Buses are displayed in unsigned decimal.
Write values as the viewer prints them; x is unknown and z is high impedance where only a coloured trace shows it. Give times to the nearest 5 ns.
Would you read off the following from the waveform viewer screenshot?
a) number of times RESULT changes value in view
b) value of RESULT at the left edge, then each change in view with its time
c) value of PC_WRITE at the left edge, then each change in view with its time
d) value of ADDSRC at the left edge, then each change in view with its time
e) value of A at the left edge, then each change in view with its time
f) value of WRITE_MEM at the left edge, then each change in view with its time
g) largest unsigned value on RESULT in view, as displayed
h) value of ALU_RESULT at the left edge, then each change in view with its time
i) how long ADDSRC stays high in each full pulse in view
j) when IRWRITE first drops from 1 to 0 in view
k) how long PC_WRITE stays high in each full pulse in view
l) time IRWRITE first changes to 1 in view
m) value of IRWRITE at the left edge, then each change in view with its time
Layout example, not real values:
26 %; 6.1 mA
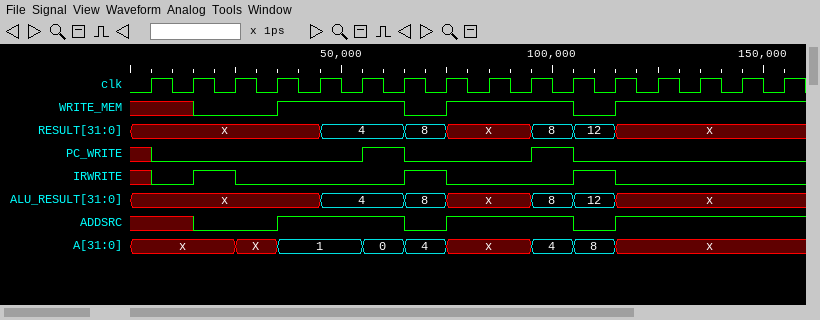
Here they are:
6; x, 4 at 45 ns, 8 at 65 ns, x at 75 ns, 8 at 95 ns, 12 at 105 ns, x at 115 ns; x, 0 at 5 ns, 1 at 55 ns, 0 at 65 ns, 1 at 95 ns, 0 at 105 ns; x, 0 at 15 ns, 1 at 35 ns, 0 at 65 ns, 1 at 75 ns, 0 at 105 ns, 1 at 115 ns; x, X at 25 ns, 1 at 35 ns, 0 at 55 ns, 4 at 65 ns, x at 75 ns, 4 at 95 ns, 8 at 105 ns, x at 115 ns; x, 0 at 15 ns, 1 at 35 ns, 0 at 65 ns, 1 at 75 ns, 0 at 105 ns, 1 at 115 ns; 12; x, 4 at 45 ns, 8 at 65 ns, x at 75 ns, 8 at 95 ns, 12 at 105 ns, x at 115 ns; 30 ns, 30 ns; 25 ns; 10 ns, 10 ns; 15 ns; x, 0 at 5 ns, 1 at 15 ns, 0 at 25 ns, 1 at 65 ns, 0 at 75 ns, 1 at 105 ns, 0 at 115 ns
